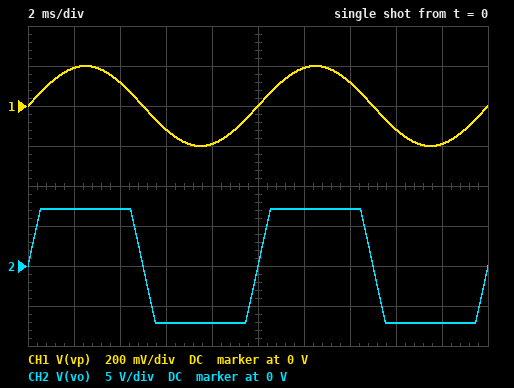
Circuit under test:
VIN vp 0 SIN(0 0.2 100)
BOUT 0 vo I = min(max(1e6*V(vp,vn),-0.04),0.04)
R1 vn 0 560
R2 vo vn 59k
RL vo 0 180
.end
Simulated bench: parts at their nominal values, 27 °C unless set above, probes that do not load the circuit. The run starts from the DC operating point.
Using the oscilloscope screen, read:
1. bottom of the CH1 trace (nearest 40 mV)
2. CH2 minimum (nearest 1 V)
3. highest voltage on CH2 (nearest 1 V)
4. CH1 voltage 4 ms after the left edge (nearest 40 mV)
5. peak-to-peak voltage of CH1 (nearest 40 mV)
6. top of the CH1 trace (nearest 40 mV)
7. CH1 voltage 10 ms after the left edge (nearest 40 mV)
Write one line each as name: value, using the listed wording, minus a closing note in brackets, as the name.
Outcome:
bottom of the CH1 trace: -200 mV
CH2 minimum: -7 V
highest voltage on CH2: 7 V
CH1 voltage 4 ms after the left edge: 120 mV
peak-to-peak voltage of CH1: 400 mV
top of the CH1 trace: 200 mV
CH1 voltage 10 ms after the left edge: 0 V
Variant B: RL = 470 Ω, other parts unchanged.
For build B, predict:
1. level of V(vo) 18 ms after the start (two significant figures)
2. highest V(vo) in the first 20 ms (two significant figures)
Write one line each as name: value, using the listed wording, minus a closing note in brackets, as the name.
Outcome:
level of V(vo) 18 ms after the start: -19 V
highest V(vo) in the first 20 ms: 19 V
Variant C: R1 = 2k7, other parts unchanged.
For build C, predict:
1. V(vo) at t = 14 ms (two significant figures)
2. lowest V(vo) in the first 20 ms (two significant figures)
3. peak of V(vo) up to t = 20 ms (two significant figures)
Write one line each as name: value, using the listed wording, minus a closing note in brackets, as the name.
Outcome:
V(vo) at t = 14 ms: 2.7 V
lowest V(vo) in the first 20 ms: -4.6 V
peak of V(vo) up to t = 20 ms: 4.6 V
